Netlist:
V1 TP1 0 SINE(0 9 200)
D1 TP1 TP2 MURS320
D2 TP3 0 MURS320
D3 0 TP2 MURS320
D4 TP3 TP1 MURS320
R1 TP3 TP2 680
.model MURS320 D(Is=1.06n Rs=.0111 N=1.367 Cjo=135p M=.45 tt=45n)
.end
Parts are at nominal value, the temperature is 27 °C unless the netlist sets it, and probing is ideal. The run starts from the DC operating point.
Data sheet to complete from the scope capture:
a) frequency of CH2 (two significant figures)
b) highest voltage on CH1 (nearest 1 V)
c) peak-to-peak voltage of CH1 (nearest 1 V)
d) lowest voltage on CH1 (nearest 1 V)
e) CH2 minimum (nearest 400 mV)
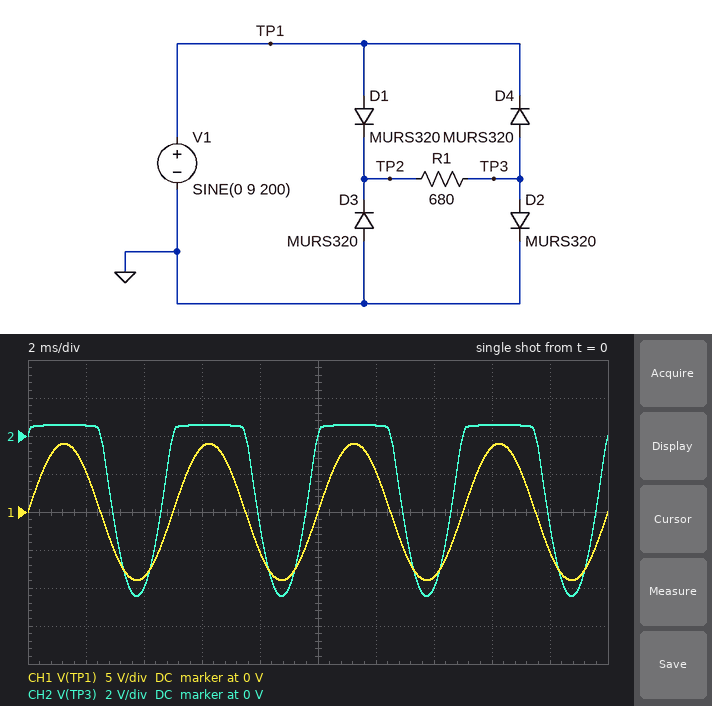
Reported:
200 Hz
9 V
18 V
-9 V
-8.4 V
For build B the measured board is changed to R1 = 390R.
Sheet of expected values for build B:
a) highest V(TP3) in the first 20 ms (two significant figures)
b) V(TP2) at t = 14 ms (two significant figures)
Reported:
590 mV
-590 mV
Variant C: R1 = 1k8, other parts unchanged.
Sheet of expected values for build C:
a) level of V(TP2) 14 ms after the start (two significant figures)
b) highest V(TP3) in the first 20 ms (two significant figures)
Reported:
-540 mV
540 mV
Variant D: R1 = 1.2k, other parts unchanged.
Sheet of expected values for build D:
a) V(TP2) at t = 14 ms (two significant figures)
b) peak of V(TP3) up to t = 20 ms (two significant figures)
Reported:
-550 mV
550 mV
